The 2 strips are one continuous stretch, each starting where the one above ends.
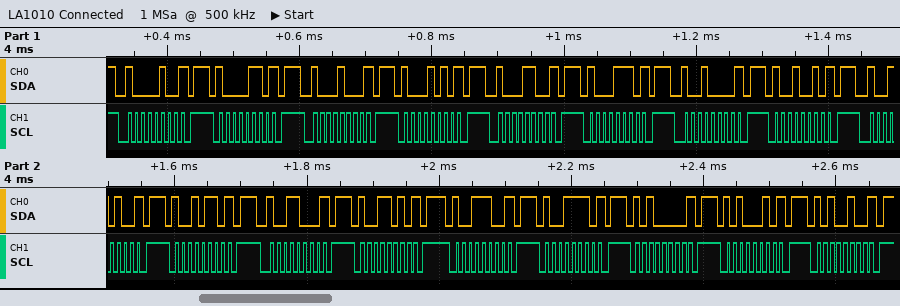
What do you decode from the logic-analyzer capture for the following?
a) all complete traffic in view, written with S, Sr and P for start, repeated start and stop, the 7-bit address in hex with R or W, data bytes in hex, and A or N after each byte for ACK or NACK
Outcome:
S 42W N P S 43W N P S 44W N P S 45W N P S 46W N P S 47W N P S 48W N P S 49W N P S 4AW N P S 4BW N P S 4CW N P S 4DW N P S 4EW N P S 4FW N P S 50W N P S 51W N P S 52W N P
